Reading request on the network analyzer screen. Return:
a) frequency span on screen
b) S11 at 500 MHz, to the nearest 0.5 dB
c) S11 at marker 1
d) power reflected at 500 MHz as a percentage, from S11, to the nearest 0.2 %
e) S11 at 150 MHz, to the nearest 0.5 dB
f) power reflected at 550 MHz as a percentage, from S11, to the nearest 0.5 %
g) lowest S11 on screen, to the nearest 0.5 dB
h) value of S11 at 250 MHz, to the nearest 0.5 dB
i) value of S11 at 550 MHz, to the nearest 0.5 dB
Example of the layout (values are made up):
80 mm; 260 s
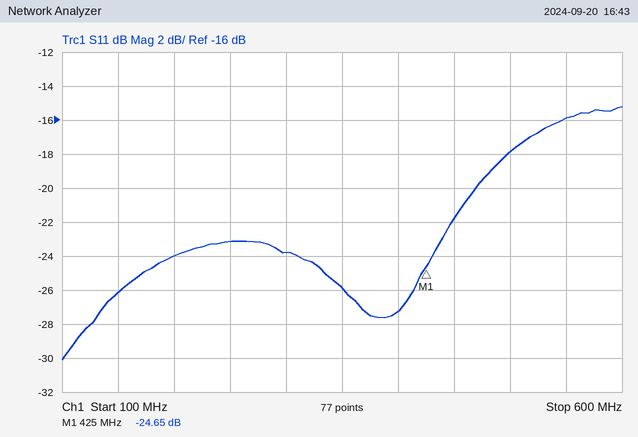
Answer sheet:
500 MHz; -18.0 dB; -24.65 dB; 1.6 %; -26.0 dB; 2.5 %; -30.0 dB; -23.0 dB; -16.0 dB
